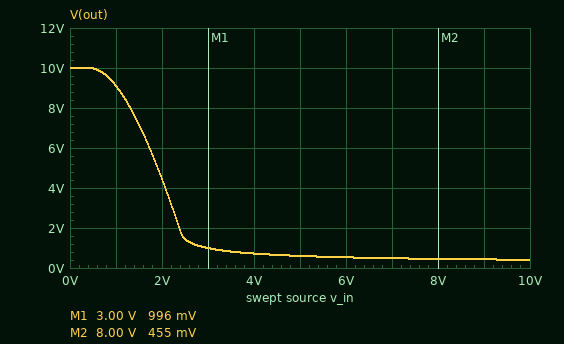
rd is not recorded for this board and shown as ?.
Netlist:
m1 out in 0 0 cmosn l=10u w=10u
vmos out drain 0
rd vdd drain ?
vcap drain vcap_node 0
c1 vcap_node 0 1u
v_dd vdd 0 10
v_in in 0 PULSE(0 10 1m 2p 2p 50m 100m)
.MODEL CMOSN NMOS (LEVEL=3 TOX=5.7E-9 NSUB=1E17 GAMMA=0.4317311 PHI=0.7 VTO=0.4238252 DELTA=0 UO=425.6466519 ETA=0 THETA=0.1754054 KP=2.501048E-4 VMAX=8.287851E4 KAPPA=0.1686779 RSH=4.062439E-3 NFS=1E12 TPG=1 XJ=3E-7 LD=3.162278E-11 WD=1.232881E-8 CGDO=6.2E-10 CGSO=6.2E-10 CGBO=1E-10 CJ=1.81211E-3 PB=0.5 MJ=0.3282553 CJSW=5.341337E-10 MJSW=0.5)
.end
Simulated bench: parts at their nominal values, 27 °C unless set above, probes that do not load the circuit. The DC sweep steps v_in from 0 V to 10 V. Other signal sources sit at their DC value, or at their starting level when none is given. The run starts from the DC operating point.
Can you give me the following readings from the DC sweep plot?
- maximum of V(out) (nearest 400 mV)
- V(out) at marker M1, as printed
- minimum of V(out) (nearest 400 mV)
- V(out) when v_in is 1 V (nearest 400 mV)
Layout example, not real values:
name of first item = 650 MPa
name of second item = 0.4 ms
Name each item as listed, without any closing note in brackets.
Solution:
maximum of V(out) = 10.0 V
V(out) at marker M1, as printed = 996 mV
minimum of V(out) = 400 mV
V(out) when v_in is 1 V = 9.2 V
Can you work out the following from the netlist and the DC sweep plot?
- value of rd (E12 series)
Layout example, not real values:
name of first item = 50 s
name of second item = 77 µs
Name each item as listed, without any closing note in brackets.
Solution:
value of rd = 27 kΩ
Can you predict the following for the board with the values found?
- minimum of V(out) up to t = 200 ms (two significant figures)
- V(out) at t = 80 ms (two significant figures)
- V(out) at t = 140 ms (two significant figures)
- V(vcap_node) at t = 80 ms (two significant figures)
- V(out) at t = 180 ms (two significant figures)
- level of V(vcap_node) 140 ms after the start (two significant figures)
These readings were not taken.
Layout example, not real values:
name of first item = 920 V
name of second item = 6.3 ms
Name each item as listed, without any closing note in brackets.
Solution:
minimum of V(out) up to t = 200 ms = 410 mV
V(out) at t = 80 ms = 6.7 V
V(out) at t = 140 ms = 410 mV
V(vcap_node) at t = 80 ms = 6.7 V
V(out) at t = 180 ms = 6.7 V
level of V(vcap_node) 140 ms after the start = 410 mV
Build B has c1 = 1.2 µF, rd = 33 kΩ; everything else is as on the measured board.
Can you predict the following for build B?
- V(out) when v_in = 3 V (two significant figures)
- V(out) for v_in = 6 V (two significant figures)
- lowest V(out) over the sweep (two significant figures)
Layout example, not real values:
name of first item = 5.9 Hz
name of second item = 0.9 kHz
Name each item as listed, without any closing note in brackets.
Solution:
V(out) when v_in = 3 V = 780 mV
V(out) for v_in = 6 V = 440 mV
lowest V(out) over the sweep = 340 mV
